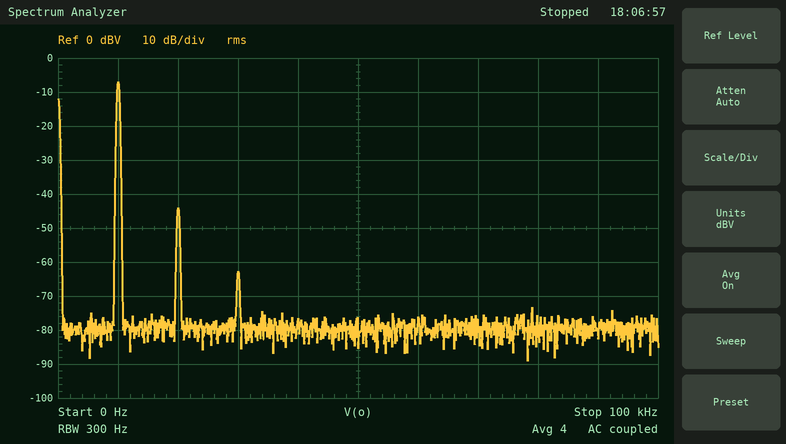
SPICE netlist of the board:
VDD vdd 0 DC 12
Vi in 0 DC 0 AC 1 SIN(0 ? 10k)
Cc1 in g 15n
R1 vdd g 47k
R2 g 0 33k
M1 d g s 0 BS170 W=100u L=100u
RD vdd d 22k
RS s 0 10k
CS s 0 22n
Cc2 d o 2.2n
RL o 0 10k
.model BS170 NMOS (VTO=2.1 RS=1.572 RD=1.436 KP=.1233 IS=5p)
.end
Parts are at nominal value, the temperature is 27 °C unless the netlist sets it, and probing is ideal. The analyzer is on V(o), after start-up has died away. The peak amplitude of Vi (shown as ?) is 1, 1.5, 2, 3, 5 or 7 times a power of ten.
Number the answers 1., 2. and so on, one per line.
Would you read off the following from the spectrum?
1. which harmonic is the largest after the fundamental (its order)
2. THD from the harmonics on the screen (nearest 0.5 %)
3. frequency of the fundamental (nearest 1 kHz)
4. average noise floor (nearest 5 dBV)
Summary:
1. 2
2. 1.5 %
3. 10 kHz
4. -80 dBV
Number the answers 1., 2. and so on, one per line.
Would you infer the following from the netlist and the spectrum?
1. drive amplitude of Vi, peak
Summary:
1. 70 mV
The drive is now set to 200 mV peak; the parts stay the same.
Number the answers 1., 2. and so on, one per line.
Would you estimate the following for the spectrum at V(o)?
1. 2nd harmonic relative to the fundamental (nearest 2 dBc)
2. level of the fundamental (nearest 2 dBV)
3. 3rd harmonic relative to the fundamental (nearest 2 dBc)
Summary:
1. -26 dBc
2. 2 dBV
3. -34 dBc
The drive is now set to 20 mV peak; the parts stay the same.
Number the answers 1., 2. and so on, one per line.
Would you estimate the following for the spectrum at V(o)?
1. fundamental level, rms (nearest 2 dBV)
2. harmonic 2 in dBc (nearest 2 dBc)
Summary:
1. -18 dBV
2. -48 dBc
